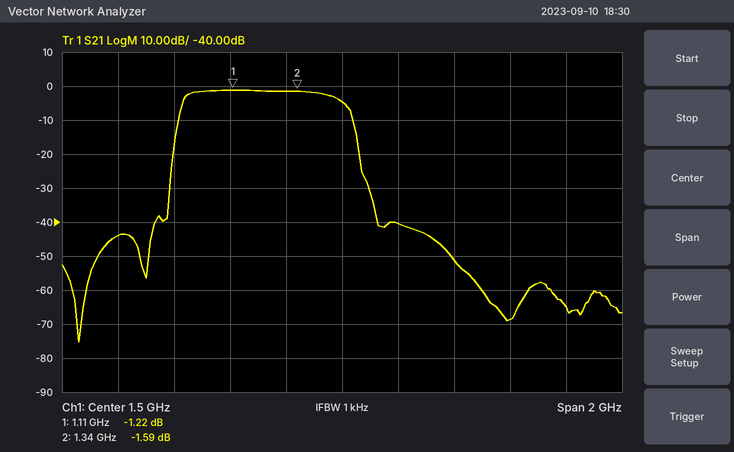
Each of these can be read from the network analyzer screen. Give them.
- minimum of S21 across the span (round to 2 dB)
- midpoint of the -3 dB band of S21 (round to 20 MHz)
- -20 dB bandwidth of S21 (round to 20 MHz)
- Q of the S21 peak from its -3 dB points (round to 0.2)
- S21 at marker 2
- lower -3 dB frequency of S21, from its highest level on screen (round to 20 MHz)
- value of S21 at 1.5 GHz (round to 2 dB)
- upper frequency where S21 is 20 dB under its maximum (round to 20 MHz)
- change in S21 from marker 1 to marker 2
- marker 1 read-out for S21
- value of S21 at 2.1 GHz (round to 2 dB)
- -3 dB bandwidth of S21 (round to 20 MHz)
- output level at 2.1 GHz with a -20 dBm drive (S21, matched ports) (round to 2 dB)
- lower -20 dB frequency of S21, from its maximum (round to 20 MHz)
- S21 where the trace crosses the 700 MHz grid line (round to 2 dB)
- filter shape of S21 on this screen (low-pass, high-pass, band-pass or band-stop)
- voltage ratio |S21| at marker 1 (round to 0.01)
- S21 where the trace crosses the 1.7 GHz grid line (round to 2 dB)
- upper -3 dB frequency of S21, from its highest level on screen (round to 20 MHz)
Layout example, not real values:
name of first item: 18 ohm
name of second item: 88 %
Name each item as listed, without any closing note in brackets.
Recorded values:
minimum of S21 across the span: -76 dB
midpoint of the -3 dB band of S21: 1.22 GHz
-20 dB bandwidth of S21: 660 MHz
Q of the S21 peak from its -3 dB points: 2.2
S21 at marker 2: -1.59 dB
lower -3 dB frequency of S21, from its highest level on screen: 940 MHz
value of S21 at 1.5 GHz: -4 dB
upper frequency where S21 is 20 dB under its maximum: 1.56 GHz
change in S21 from marker 1 to marker 2: -0.37 dB
marker 1 read-out for S21: -1.22 dB
value of S21 at 2.1 GHz: -68 dB
-3 dB bandwidth of S21: 560 MHz
output level at 2.1 GHz with a -20 dBm drive (S21, matched ports): -88 dBm
lower -20 dB frequency of S21, from its maximum: 900 MHz
S21 where the trace crosses the 700 MHz grid line: -44 dB
filter shape of S21 on this screen: band-pass
voltage ratio |S21| at marker 1: 0.87
S21 where the trace crosses the 1.7 GHz grid line: -40 dB
upper -3 dB frequency of S21, from its highest level on screen: 1.50 GHz
